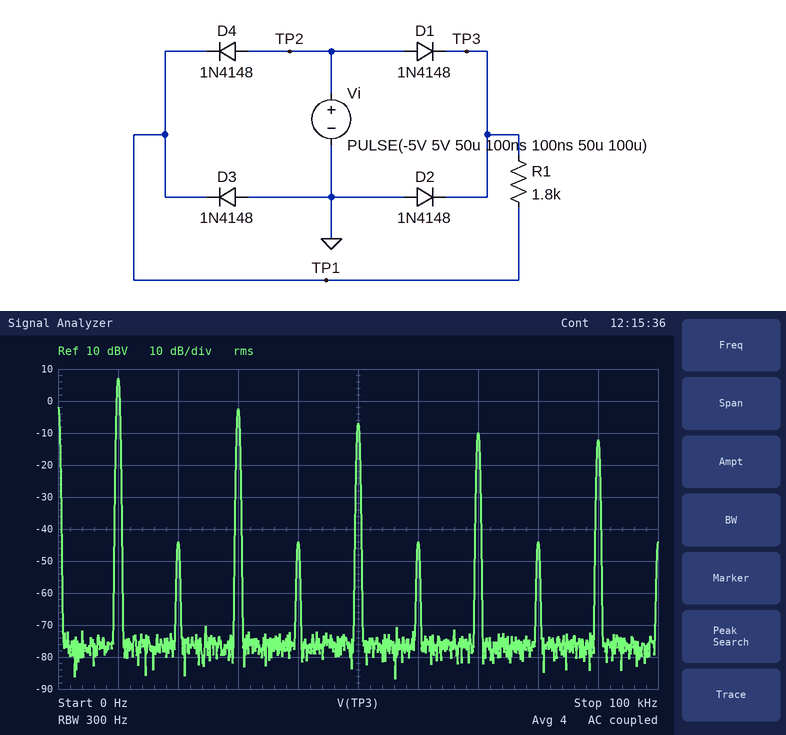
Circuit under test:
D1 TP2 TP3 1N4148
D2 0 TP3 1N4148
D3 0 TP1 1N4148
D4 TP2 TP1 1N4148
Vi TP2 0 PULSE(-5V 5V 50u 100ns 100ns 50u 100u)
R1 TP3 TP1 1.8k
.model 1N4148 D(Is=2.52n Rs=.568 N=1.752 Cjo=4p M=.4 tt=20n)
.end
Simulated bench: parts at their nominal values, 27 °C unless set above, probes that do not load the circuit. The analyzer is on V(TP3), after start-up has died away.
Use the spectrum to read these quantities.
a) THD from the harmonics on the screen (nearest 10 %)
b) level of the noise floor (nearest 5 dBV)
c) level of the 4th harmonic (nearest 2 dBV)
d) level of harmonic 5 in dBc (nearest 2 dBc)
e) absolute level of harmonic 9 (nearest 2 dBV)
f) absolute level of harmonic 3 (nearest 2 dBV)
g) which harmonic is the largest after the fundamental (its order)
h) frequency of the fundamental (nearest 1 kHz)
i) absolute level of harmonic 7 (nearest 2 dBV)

40 %
-75 dBV
-44 dBV
-14 dBc
-12 dBV
-2 dBV
3
10 kHz
-10 dBV
